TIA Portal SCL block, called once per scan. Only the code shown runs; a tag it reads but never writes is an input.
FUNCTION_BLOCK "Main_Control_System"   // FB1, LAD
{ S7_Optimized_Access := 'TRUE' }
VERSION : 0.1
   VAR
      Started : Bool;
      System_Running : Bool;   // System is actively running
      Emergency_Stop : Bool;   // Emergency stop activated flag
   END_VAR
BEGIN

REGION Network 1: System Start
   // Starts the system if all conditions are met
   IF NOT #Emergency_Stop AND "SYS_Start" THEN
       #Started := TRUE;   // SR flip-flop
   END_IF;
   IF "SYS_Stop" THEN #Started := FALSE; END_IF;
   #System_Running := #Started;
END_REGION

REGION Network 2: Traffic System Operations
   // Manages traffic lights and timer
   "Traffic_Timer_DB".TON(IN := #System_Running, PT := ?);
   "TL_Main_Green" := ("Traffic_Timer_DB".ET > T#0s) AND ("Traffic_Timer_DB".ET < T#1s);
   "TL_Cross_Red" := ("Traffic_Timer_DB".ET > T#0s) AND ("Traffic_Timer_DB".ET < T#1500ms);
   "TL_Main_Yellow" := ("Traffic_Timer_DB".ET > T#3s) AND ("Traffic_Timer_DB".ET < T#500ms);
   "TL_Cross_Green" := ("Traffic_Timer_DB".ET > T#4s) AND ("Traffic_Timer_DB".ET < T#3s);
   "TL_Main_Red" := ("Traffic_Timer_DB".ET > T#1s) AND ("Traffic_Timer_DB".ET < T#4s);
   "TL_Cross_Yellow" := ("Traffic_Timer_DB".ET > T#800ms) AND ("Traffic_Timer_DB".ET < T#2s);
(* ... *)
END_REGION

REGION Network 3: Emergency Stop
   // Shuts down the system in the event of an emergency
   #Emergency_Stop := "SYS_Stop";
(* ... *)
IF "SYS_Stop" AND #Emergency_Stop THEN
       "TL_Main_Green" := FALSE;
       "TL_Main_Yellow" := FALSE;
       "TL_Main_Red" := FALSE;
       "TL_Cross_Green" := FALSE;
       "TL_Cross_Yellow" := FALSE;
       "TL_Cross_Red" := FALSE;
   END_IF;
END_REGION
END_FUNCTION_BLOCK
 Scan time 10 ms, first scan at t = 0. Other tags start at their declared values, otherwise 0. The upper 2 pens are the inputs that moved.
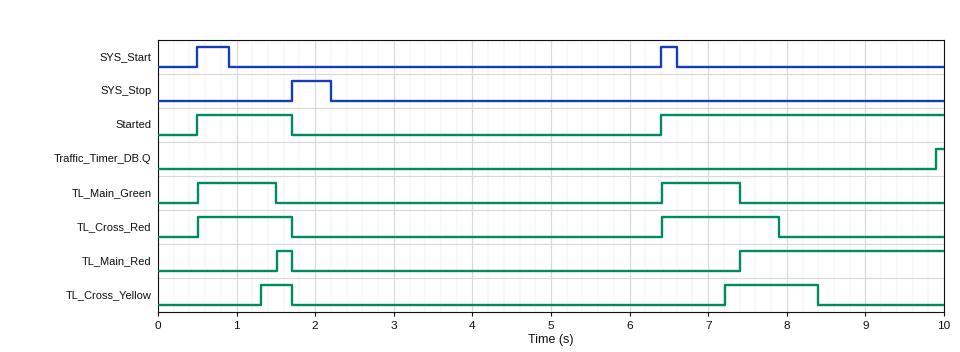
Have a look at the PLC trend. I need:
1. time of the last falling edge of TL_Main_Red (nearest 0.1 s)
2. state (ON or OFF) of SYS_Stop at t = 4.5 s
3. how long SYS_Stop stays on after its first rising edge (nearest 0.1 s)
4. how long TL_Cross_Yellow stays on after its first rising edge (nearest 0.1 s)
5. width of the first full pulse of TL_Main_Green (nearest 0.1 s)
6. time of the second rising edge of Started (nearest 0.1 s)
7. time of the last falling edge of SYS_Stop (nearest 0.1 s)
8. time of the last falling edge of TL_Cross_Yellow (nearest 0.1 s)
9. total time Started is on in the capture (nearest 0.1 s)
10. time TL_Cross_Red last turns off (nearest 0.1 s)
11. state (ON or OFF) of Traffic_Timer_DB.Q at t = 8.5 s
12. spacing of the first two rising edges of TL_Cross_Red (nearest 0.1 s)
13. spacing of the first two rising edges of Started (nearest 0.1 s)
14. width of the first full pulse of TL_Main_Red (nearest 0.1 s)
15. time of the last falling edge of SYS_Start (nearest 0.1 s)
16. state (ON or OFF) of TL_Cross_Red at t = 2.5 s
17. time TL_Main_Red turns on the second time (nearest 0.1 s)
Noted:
1.7 s
OFF
0.5 s
0.4 s
1.0 s
6.4 s
2.2 s
8.4 s
4.8 s
7.9 s
OFF
5.9 s
5.9 s
0.2 s
6.6 s
OFF
7.4 s
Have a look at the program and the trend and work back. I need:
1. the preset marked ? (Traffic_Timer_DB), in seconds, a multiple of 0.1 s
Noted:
3.5 s
